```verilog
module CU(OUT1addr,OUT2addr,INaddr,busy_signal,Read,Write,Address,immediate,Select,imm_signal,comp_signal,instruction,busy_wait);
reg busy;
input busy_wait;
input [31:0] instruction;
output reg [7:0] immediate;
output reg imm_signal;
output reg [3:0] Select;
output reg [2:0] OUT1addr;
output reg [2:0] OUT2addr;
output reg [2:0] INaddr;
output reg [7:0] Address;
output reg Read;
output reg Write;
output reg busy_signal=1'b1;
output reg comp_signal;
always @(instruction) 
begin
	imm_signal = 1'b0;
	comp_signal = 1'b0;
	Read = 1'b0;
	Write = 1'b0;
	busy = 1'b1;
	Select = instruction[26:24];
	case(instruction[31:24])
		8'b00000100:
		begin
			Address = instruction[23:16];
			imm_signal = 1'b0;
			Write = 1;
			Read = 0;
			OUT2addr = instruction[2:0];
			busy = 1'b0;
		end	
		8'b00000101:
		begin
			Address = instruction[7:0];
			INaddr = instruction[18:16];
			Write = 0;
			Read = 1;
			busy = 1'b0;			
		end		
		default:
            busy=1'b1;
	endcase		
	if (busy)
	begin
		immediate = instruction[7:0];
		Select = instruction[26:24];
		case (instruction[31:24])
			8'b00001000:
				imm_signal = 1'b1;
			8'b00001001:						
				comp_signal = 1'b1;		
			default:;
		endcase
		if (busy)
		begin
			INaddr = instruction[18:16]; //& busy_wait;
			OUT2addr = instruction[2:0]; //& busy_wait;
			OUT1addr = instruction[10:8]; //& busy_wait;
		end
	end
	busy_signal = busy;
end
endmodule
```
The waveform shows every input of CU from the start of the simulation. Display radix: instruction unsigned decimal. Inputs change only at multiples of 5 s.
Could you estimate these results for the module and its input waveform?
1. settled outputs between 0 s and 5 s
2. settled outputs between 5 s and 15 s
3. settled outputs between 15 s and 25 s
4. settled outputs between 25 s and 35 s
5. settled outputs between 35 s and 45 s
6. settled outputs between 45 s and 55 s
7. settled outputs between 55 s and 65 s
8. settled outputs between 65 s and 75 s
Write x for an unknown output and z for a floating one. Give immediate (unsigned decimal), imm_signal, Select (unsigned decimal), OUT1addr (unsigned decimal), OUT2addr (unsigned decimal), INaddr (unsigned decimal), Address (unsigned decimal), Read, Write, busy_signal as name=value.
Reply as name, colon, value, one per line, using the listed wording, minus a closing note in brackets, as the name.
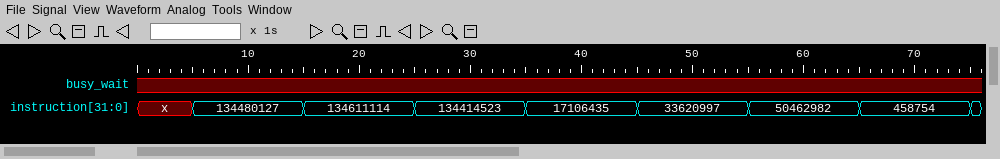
settled outputs between 0 s and 5 s: immediate=x, imm_signal=x, Select=x, OUT1addr=x, OUT2addr=x, INaddr=x, Address=x, Read=x, Write=x, busy_signal=1
settled outputs between 5 s and 15 s: immediate=255, imm_signal=1, Select=0, OUT1addr=0, OUT2addr=7, INaddr=4, Address=x, Read=0, Write=0, busy_signal=1
settled outputs between 15 s and 25 s: immediate=170, imm_signal=1, Select=0, OUT1addr=0, OUT2addr=2, INaddr=6, Address=x, Read=0, Write=0, busy_signal=1
settled outputs between 25 s and 35 s: immediate=187, imm_signal=1, Select=0, OUT1addr=0, OUT2addr=3, INaddr=3, Address=x, Read=0, Write=0, busy_signal=1
settled outputs between 35 s and 45 s: immediate=3, imm_signal=0, Select=1, OUT1addr=6, OUT2addr=3, INaddr=5, Address=x, Read=0, Write=0, busy_signal=1
settled outputs between 45 s and 55 s: immediate=5, imm_signal=0, Select=2, OUT1addr=4, OUT2addr=5, INaddr=1, Address=x, Read=0, Write=0, busy_signal=1
settled outputs between 55 s and 65 s: immediate=6, imm_signal=0, Select=3, OUT1addr=1, OUT2addr=6, INaddr=2, Address=x, Read=0, Write=0, busy_signal=1
settled outputs between 65 s and 75 s: immediate=2, imm_signal=0, Select=0, OUT1addr=0, OUT2addr=2, INaddr=7, Address=x, Read=0, Write=0, busy_signal=1
